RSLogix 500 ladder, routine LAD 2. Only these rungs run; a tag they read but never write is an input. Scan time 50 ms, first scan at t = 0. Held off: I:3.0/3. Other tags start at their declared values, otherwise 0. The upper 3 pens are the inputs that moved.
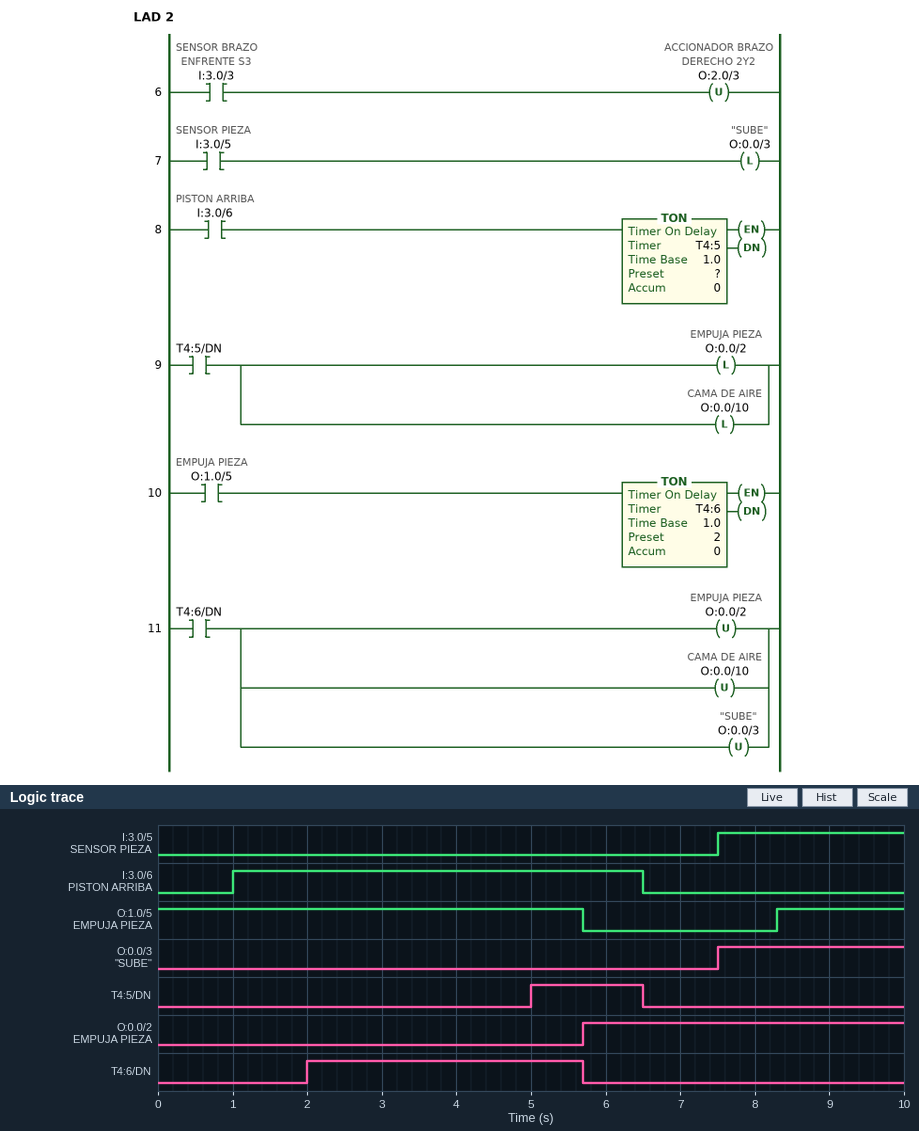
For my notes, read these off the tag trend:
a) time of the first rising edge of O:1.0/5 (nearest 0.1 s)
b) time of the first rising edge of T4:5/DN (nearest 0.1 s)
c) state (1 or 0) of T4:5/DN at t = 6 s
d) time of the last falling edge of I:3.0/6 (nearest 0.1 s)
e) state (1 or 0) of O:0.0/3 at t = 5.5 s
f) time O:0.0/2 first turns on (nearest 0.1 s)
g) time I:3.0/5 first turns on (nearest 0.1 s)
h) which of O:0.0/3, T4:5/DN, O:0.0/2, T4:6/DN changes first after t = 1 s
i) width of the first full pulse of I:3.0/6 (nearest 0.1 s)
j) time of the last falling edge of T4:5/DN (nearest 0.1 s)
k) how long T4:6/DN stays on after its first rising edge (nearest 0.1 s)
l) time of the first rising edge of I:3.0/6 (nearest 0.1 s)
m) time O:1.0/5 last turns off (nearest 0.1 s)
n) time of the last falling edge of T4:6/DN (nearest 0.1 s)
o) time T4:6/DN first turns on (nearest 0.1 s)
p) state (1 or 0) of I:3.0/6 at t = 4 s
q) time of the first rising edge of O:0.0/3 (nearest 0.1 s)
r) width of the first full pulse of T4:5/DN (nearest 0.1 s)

8.3 s
5.0 s
1
6.5 s
0
5.7 s
7.5 s
T4:6/DN
5.5 s
6.5 s
3.7 s
1.0 s
5.7 s
5.7 s
2.0 s
1
7.5 s
1.5 s
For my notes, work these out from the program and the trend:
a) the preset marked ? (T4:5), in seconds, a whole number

4 s
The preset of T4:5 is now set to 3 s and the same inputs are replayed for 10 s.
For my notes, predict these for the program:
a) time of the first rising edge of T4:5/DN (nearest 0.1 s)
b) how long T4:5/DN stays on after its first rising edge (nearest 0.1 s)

4.0 s
2.5 s
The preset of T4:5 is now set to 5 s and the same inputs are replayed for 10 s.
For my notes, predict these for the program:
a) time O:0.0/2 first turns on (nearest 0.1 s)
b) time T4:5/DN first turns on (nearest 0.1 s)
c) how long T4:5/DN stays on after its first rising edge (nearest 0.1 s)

6.0 s
6.0 s
0.5 s
